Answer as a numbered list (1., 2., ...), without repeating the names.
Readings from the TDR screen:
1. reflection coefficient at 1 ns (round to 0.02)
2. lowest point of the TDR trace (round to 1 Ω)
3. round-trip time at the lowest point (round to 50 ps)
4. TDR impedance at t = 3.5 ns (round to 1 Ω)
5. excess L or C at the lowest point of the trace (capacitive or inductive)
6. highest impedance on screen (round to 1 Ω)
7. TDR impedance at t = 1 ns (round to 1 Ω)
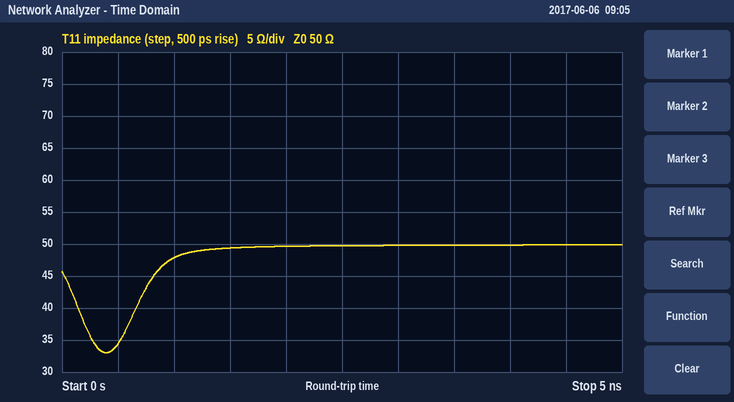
1. -0.02
2. 33 Ω
3. 400 ps
4. 50 Ω
5. capacitive
6. 50 Ω
7. 48 Ω
